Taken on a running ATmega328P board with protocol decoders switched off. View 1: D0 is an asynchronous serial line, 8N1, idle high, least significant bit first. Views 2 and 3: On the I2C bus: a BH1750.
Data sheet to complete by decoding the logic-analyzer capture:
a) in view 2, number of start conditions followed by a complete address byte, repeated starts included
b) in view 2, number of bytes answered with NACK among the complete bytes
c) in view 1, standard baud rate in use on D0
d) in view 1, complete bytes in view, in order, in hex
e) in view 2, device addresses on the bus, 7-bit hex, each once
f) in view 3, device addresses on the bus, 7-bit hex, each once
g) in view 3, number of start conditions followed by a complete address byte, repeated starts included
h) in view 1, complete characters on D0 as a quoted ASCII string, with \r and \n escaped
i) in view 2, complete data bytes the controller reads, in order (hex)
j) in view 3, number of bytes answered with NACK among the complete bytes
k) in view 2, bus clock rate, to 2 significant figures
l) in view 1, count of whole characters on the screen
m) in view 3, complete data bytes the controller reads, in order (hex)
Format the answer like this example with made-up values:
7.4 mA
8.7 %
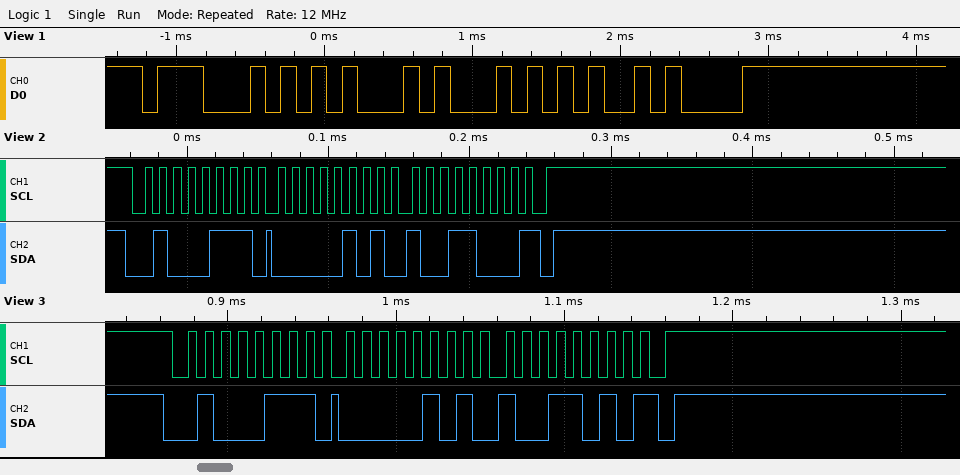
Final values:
1
1
9600 baud
47 45 54 0A
0x23
0x23
1
"GET\n"
05 98
1
100 kHz
4
05 9A
